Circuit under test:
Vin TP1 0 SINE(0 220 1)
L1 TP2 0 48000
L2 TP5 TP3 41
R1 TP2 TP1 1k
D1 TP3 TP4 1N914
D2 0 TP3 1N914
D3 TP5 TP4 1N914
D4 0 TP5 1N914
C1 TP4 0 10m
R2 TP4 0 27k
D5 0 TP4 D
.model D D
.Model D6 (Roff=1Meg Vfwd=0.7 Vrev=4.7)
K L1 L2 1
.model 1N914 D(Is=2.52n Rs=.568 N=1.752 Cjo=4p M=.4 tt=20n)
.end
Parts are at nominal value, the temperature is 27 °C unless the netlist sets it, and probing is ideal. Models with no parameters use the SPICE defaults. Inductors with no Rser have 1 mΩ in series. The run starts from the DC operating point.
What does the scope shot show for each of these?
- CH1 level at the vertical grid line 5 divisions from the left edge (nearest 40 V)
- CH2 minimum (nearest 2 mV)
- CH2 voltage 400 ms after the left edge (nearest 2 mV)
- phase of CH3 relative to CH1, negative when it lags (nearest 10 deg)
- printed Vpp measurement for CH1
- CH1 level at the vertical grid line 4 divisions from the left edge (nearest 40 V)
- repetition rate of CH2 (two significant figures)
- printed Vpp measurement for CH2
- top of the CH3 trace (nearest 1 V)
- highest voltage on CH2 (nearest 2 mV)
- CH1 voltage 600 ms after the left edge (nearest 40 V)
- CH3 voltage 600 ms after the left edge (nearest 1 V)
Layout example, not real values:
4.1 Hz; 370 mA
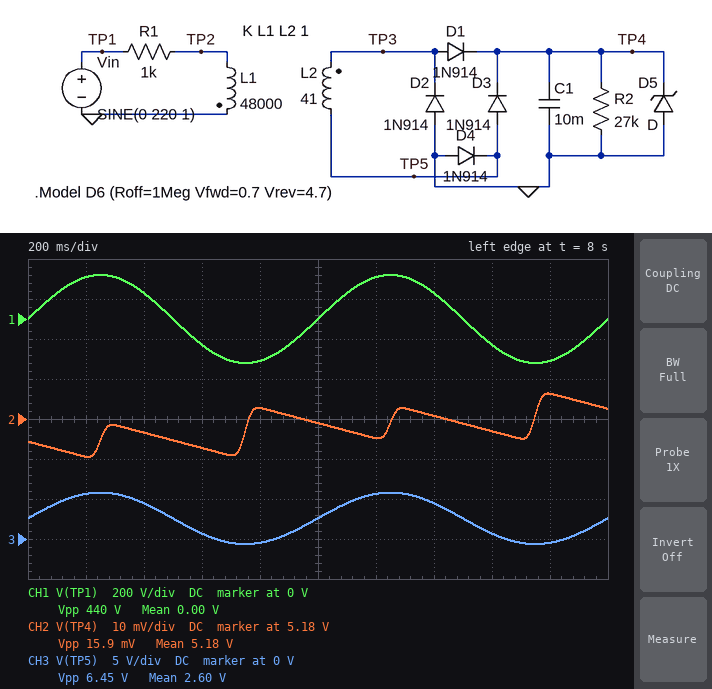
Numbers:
0 V; 5.170 V; 5.176 V; 0 deg; 440 V; -200 V; 2.1 Hz; 15.9 mV; 6 V; 5.186 V; -120 V; 1 V
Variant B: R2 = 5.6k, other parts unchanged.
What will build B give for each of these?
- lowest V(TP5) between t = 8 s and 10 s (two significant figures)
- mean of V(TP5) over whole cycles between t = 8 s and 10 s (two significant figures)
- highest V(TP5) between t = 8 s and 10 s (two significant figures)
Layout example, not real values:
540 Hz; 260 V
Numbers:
-700 mV; 2.5 V; 5.7 V
